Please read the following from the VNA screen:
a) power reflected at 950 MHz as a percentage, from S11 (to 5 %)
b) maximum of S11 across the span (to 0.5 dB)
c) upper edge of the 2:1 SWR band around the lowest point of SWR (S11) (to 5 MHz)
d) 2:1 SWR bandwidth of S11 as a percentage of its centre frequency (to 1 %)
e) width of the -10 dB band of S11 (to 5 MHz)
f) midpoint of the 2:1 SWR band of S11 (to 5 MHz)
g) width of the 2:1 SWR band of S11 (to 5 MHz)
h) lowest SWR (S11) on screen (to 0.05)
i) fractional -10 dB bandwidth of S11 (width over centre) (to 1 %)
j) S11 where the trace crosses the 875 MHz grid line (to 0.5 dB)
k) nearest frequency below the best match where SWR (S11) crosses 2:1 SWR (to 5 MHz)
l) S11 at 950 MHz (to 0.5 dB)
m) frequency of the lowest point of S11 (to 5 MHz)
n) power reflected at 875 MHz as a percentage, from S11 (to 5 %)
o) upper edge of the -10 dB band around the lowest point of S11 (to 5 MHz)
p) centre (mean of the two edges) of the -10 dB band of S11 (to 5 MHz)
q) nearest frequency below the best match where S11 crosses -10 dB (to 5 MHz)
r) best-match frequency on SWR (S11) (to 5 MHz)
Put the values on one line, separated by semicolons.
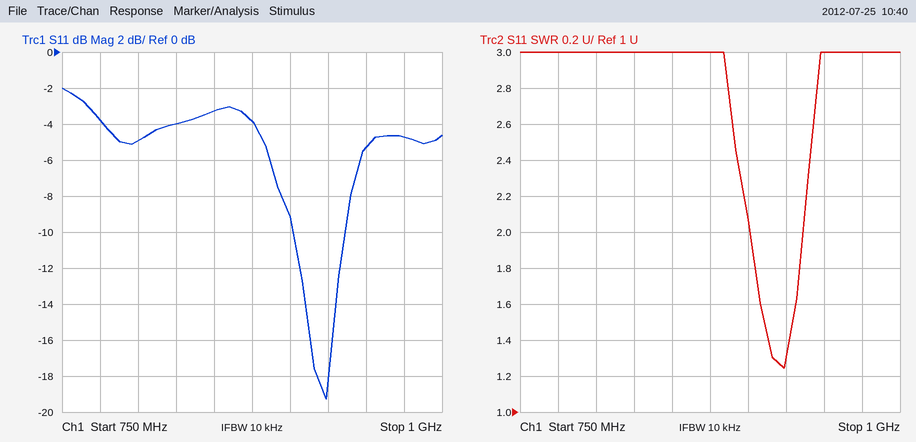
30 %; -2.0 dB; 935 MHz; 4 %; 35 MHz; 920 MHz; 35 MHz; 1.25; 4 %; -4.0 dB; 900 MHz; -5.5 dB; 925 MHz; 40 %; 935 MHz; 920 MHz; 900 MHz; 925 MHz
